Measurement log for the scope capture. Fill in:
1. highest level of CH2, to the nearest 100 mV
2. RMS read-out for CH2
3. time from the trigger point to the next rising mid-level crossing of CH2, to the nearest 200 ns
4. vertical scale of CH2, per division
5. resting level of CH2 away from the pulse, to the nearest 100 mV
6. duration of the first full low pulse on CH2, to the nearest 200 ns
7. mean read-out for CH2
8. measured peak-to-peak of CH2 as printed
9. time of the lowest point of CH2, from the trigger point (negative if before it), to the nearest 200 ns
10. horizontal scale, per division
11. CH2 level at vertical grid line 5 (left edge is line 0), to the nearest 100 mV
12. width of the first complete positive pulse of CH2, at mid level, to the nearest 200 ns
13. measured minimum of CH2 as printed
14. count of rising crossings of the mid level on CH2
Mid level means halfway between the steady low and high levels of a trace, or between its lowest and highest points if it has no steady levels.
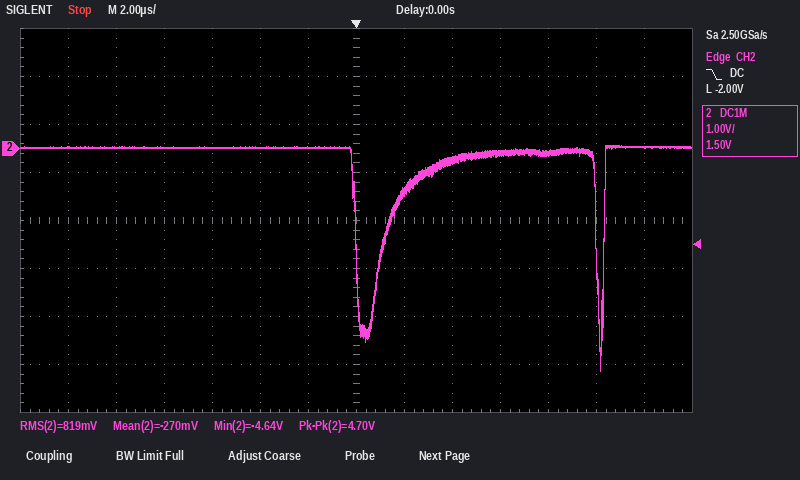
100 mV
819 mV
1.0 µs
1 V
0.0 V
1.0 µs
-270 mV
4.70 V
+10.2 µs
2 µs
0.0 V
9.0 µs
-4.64 V
2
